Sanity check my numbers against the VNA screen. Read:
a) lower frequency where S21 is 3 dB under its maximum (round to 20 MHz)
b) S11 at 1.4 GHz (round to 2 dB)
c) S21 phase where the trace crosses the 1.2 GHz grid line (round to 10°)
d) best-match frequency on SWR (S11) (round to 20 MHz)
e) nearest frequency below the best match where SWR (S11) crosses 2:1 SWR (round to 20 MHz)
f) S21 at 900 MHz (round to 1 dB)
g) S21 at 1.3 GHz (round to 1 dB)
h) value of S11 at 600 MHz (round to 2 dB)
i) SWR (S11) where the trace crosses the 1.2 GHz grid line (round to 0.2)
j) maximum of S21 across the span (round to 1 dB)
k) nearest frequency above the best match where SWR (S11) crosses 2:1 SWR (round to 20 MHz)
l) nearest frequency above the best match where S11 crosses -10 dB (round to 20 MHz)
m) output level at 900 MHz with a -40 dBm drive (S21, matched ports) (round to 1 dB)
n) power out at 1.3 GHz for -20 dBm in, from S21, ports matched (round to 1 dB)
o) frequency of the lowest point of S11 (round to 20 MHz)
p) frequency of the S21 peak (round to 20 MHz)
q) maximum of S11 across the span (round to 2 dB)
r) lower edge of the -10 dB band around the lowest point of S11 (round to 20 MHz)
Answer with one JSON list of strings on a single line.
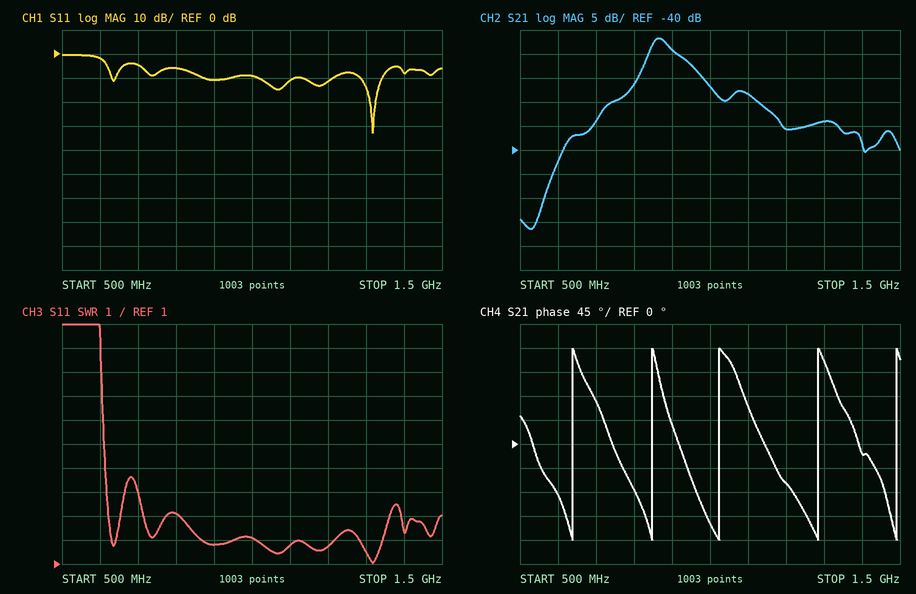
["840 MHz", "-8 dB", "-70°", "1.32 GHz", "1.28 GHz", "-19 dB", "-34 dB", "-2 dB", "1.8", "-17 dB", "1.34 GHz", "1.34 GHz", "-59 dBm", "-54 dBm", "1.32 GHz", "860 MHz", "0 dB", "1.28 GHz"]
